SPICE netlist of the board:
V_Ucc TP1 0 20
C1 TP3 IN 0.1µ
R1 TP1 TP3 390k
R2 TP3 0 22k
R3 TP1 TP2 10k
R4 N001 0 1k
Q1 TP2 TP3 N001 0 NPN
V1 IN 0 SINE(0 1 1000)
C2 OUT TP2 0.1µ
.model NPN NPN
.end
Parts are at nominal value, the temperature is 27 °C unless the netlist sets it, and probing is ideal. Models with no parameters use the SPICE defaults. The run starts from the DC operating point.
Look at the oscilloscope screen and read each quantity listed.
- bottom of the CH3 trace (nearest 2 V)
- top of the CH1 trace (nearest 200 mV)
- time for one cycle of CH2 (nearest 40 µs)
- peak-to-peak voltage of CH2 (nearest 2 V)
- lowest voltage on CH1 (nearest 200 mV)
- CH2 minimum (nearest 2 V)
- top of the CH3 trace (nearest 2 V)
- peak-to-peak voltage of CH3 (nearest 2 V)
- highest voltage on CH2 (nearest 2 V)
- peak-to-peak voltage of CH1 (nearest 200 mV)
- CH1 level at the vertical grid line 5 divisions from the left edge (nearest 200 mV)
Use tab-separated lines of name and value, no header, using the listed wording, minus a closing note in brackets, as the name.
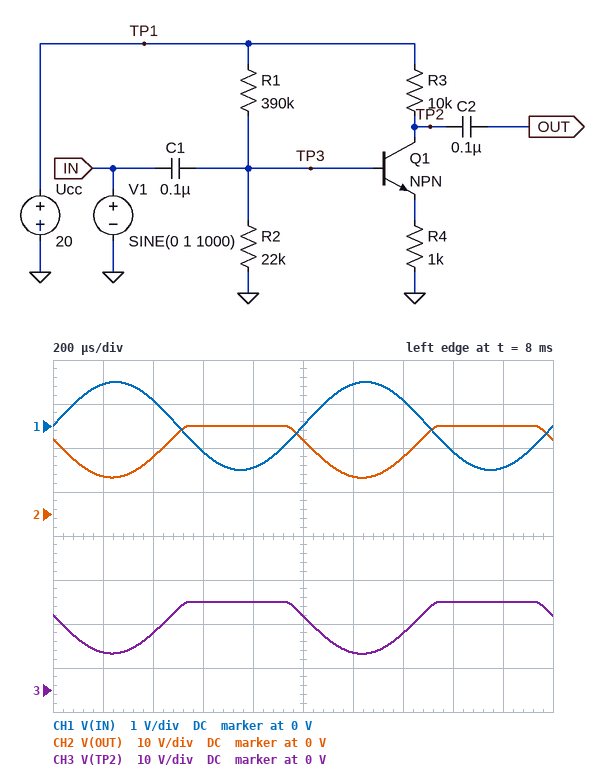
bottom of the CH3 trace	8 V
top of the CH1 trace	1.0 V
time for one cycle of CH2	1.00 ms
peak-to-peak voltage of CH2	12 V
lowest voltage on CH1	-1.0 V
CH2 minimum	8 V
top of the CH3 trace	20 V
peak-to-peak voltage of CH3	12 V
highest voltage on CH2	20 V
peak-to-peak voltage of CH1	2.0 V
CH1 level at the vertical grid line 5 divisions from the left edge	0 V
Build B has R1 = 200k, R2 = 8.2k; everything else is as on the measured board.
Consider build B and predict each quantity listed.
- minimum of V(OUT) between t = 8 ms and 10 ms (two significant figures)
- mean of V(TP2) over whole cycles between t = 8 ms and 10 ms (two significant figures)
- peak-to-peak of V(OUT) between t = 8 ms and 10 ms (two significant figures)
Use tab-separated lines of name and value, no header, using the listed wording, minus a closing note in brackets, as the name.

minimum of V(OUT) between t = 8 ms and 10 ms	10 V
mean of V(TP2) over whole cycles between t = 8 ms and 10 ms	17 V
peak-to-peak of V(OUT) between t = 8 ms and 10 ms	9.6 V
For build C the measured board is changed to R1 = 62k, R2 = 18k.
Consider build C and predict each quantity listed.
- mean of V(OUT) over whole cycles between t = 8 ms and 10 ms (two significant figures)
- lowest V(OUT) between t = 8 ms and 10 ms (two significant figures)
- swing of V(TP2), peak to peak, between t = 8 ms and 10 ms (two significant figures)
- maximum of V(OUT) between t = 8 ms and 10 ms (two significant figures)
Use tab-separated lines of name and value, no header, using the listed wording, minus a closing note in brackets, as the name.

mean of V(OUT) over whole cycles between t = 8 ms and 10 ms	6.0 V
lowest V(OUT) between t = 8 ms and 10 ms	2.0 V
swing of V(TP2), peak to peak, between t = 8 ms and 10 ms	11 V
maximum of V(OUT) between t = 8 ms and 10 ms	13 V
